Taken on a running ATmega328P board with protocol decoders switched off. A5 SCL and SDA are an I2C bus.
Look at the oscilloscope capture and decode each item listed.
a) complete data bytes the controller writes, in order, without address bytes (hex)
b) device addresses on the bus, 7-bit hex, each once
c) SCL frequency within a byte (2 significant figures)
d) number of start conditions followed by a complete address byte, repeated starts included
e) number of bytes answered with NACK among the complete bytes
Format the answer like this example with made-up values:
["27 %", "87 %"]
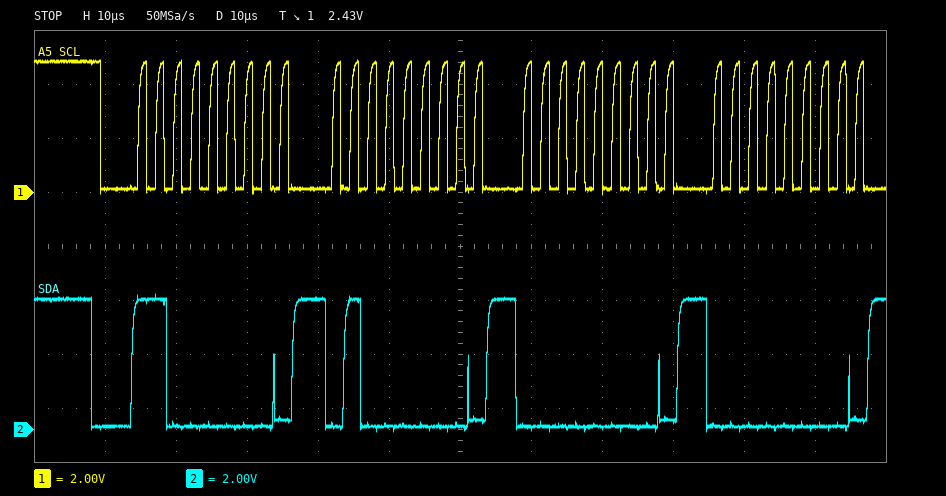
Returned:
["40 00 00", "0x60", "400 kHz", "1", "0"]
